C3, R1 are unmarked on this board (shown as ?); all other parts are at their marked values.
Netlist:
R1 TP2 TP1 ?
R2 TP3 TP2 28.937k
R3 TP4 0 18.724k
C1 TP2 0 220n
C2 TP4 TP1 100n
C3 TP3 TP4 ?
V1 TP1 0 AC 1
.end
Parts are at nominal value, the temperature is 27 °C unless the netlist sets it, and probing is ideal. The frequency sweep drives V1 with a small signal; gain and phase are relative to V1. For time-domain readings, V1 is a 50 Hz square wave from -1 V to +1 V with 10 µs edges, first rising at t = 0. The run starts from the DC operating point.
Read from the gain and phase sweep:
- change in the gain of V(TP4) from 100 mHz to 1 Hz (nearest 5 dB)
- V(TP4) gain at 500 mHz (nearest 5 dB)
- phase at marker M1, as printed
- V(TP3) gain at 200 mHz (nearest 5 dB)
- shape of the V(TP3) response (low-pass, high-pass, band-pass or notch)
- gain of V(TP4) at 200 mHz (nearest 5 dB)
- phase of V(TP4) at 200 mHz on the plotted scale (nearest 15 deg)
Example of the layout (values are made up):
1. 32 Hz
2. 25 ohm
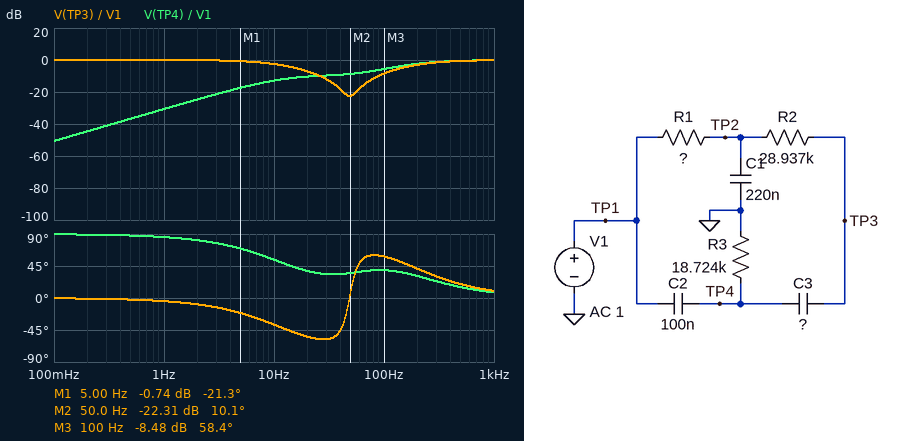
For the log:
1. 20 dB
2. -35 dB
3. -21.3 deg
4. 0 dB
5. notch
6. -45 dB
7. 90 deg
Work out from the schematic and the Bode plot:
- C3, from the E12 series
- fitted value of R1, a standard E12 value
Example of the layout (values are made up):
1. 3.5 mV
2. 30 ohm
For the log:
1. 150 nF
2. 22 kΩ
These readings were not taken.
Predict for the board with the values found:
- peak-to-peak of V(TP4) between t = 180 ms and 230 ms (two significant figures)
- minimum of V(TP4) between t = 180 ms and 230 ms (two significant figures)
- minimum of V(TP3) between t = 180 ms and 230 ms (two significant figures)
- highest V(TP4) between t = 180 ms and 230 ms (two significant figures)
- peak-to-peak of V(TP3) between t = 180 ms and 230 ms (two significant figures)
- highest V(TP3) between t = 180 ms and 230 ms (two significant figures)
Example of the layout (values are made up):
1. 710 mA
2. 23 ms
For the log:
1. 3.6 V
2. -1.8 V
3. -1.6 V
4. 1.8 V
5. 3.3 V
6. 1.6 V
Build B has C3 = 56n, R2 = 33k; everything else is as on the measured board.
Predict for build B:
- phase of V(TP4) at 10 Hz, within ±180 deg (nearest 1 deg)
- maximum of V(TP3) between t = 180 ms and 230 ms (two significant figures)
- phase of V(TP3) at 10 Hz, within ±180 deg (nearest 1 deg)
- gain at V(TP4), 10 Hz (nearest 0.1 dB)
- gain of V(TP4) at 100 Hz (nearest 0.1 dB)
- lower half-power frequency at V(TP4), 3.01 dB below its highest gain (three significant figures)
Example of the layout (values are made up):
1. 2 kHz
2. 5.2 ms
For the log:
1. 71 deg
2. 1.5 V
3. -27 deg
4. -15.4 dB
5. -4.6 dB
6. 156 Hz
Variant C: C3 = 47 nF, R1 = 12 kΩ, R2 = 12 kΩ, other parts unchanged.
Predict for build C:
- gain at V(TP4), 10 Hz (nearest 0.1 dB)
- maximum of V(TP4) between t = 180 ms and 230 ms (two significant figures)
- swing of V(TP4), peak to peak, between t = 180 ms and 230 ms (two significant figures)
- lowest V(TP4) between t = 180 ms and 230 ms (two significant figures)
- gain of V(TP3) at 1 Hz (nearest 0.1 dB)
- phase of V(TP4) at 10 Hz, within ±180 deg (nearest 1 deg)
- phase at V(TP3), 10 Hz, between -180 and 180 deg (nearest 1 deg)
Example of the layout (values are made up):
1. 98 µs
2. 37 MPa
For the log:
1. -15.5 dB
2. 1.9 V
3. 3.8 V
4. -1.9 V
5. 0 dB
6. 76 deg
7. -13 deg
